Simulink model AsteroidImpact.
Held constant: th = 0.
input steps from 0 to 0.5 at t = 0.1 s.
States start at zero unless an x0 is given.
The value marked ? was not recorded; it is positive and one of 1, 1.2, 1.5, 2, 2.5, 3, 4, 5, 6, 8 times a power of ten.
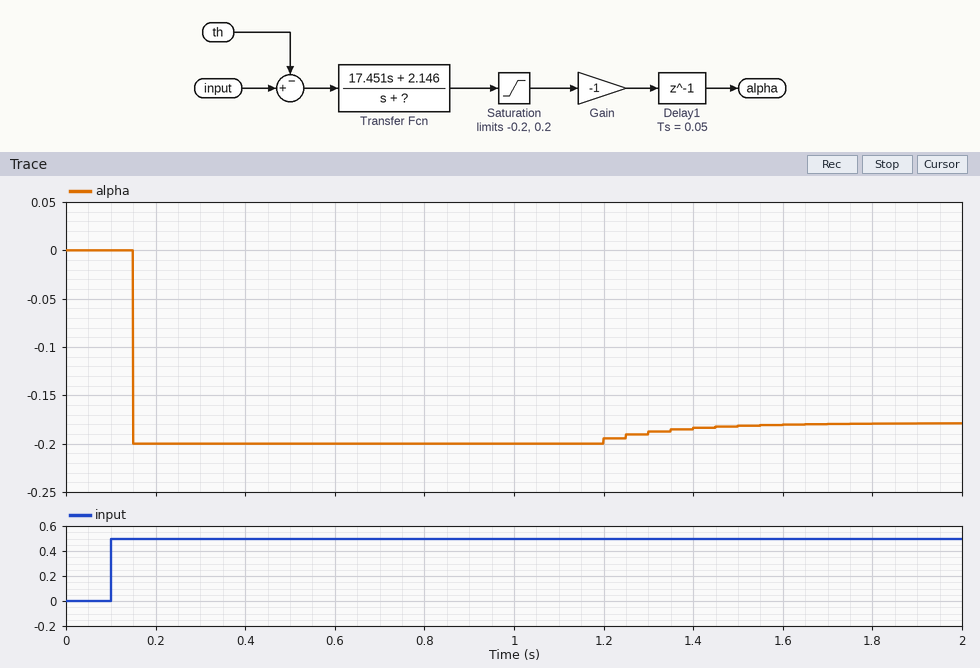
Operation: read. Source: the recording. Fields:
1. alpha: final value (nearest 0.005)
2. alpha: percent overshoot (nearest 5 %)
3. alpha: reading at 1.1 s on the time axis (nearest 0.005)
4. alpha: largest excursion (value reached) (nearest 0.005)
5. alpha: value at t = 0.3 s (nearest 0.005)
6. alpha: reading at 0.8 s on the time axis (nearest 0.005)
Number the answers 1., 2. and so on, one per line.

1. -0.180
2. 10 %
3. -0.200
4. -0.200
5. -0.200
6. -0.200
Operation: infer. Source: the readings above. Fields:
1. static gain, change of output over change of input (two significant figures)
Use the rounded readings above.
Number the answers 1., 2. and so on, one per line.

1. -0.36
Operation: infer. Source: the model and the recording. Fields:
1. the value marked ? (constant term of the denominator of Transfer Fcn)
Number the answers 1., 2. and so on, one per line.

1. 6
